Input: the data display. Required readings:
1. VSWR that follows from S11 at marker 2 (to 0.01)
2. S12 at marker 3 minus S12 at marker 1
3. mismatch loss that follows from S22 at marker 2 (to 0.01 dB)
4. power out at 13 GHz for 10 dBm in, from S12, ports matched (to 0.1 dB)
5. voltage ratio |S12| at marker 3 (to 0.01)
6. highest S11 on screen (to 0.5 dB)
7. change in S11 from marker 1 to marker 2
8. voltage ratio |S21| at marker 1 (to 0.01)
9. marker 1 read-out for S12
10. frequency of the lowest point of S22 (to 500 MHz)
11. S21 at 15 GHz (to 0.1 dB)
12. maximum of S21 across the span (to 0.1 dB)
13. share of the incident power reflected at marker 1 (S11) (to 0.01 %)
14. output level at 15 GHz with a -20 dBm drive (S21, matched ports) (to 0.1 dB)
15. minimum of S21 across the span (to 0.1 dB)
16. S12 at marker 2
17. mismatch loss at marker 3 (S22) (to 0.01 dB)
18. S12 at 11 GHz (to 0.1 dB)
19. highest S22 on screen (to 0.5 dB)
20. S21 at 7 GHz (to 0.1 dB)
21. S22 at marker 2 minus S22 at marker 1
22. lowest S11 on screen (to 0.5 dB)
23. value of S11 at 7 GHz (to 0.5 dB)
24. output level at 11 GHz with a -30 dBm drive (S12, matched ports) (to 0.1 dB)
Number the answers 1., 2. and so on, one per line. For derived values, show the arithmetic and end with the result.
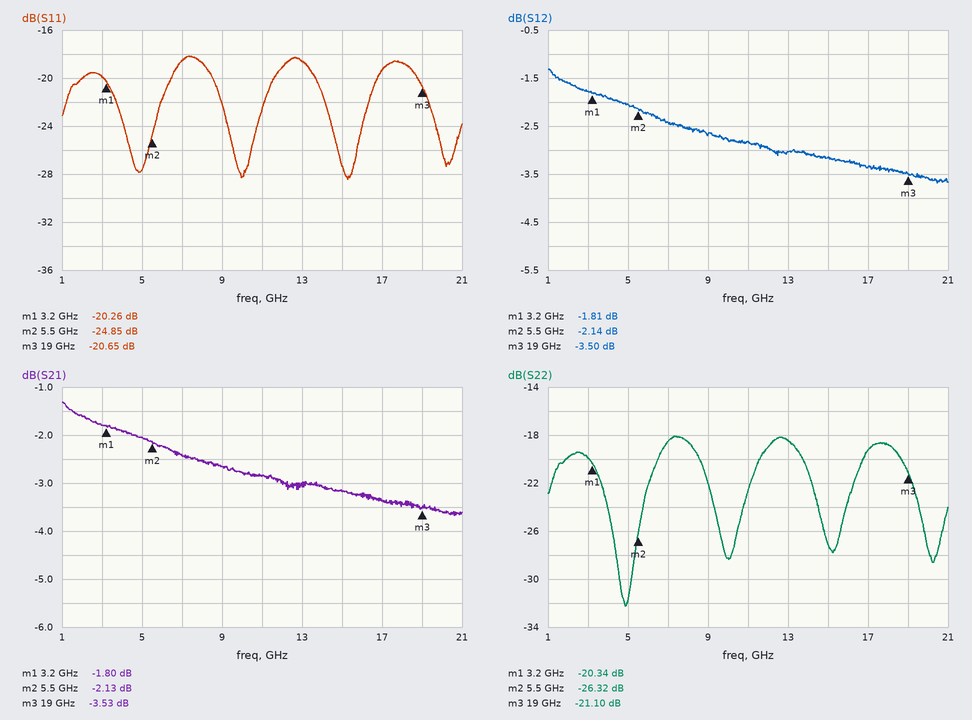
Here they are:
1. (1 + 0.0572)/(1 − 0.0572) ≈ 1.12
2. -3.5 − (-1.81) = -1.69 dB
3. −10 log10(1 − 10^(-26.32/10)) ≈ 0.01 dB
4. 10 dBm + (-3.0 dB) = 7.0 dBm
5. 10^(-3.5/20) ≈ 0.67
6. -18.0 dB
7. -24.85 − (-20.26) = -4.59 dB
8. 10^(-1.8/20) ≈ 0.81
9. -1.81 dB
10. 5.0 GHz
11. -3.2 dB
12. -1.3 dB
13. 10^(-20.26/10) ≈ 0.94 %
14. -20 dBm + (-3.2 dB) = -23.2 dBm
15. -3.7 dB
16. -2.14 dB
17. −10 log10(1 − 10^(-21.1/10)) ≈ 0.03 dB
18. -2.8 dB
19. -18.0 dB
20. -2.4 dB
21. -26.32 − (-20.34) = -5.98 dB
22. -28.5 dB
23. -18.5 dB
24. -30 dBm + (-2.8 dB) = -32.8 dBm
